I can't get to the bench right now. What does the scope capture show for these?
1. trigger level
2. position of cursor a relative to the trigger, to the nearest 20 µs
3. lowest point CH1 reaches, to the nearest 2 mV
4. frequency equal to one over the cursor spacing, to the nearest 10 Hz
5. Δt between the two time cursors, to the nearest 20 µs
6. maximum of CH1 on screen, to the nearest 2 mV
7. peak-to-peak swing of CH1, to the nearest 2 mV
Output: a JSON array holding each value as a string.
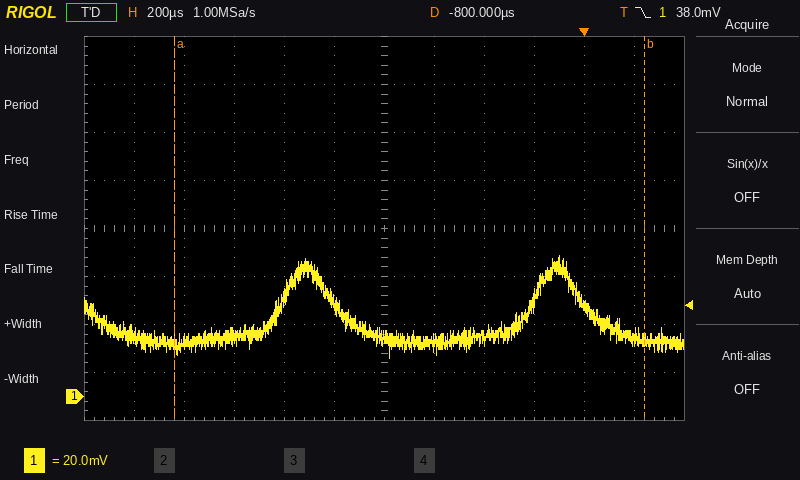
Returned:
["38.0 mV", "-1.64 ms", "16 mV", "530 Hz", "1.88 ms", "58 mV", "42 mV"]
